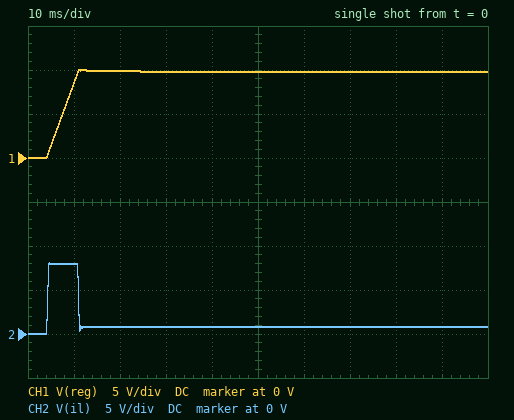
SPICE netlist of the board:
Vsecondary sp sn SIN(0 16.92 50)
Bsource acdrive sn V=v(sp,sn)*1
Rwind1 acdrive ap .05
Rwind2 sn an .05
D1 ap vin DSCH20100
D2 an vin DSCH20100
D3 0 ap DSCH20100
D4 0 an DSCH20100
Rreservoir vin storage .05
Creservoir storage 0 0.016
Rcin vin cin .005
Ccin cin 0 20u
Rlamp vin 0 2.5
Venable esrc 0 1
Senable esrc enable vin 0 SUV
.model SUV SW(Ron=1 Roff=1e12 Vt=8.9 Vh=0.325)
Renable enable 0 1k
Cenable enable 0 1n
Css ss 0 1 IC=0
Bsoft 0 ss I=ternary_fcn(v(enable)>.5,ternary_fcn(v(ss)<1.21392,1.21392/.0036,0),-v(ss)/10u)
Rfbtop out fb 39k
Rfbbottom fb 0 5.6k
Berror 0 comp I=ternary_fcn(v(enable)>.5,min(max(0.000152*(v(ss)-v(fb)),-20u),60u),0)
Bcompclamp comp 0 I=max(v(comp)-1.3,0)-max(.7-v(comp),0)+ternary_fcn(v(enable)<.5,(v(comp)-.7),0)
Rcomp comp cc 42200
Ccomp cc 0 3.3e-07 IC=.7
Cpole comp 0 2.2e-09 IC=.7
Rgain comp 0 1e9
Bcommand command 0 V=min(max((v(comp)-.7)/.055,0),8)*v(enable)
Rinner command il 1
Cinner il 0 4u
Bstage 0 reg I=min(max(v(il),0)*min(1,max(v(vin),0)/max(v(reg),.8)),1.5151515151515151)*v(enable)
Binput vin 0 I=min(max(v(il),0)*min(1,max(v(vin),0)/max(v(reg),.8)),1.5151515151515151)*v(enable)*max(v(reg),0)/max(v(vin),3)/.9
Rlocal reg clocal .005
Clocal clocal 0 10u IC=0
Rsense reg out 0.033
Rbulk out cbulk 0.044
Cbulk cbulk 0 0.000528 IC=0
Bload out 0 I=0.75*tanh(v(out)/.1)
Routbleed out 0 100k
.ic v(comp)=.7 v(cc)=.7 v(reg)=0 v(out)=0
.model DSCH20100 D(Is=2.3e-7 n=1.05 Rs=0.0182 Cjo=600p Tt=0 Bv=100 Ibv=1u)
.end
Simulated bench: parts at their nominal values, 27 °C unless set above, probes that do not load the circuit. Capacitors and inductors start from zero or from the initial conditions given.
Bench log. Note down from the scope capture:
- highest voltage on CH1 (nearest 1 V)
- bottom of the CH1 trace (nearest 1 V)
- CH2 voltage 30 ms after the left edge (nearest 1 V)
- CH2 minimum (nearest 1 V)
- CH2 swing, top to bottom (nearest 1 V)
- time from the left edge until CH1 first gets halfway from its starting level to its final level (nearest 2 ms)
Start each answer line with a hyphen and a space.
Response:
- 10 V
- 0 V
- 1 V
- 0 V
- 8 V
- 8 ms
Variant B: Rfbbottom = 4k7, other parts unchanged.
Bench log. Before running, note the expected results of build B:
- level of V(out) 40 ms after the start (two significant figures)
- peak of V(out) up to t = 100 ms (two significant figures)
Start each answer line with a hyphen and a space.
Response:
- 11 V
- 12 V
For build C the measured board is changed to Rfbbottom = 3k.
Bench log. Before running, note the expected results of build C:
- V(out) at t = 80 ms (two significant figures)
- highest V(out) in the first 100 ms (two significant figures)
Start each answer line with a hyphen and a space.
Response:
- 17 V
- 18 V
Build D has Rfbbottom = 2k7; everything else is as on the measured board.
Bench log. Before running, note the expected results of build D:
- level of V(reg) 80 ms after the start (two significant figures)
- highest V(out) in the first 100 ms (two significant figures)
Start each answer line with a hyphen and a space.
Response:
- 19 V
- 20 V
